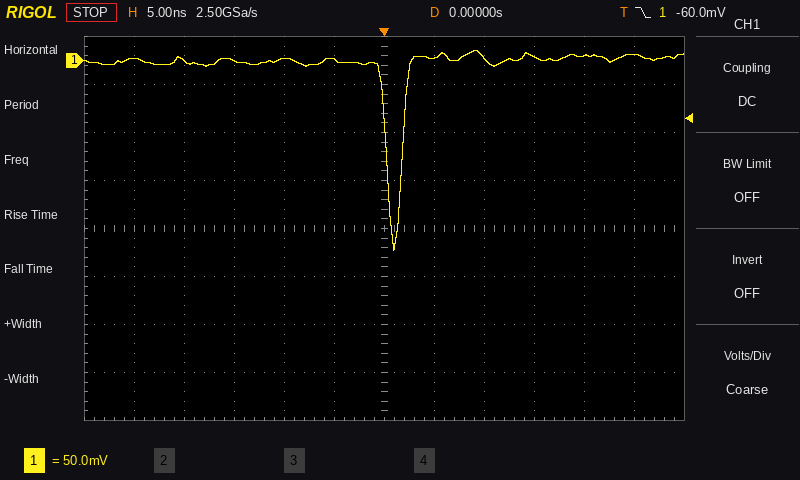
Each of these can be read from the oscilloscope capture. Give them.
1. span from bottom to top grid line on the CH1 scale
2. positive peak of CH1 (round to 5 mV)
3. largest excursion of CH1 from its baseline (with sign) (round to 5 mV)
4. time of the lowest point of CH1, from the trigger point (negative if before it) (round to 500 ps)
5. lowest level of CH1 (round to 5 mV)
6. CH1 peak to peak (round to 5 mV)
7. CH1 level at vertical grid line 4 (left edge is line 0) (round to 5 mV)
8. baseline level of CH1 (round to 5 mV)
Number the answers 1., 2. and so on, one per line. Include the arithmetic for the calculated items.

1. 400 mV
2. 10 mV
3. -200 mV − (0 mV) = -200 mV
4. +1.0 ns
5. -200 mV
6. 10 mV − (-200 mV) = 210 mV
7. 0 mV
8. 0 mV
